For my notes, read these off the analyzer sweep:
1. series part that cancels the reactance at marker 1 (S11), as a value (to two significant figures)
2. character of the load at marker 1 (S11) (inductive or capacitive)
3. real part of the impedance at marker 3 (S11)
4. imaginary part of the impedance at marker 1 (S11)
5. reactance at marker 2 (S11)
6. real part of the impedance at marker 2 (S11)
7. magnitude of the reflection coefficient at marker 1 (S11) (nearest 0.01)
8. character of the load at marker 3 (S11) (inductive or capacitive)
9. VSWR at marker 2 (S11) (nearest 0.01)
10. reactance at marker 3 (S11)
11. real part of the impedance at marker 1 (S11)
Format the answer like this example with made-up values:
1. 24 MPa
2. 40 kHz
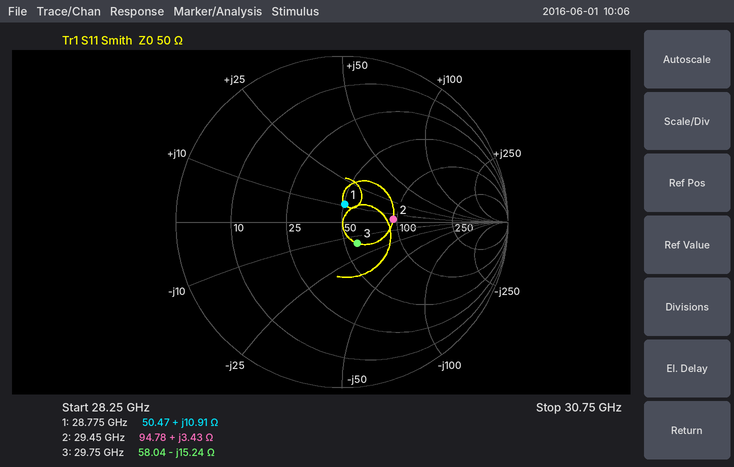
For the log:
1. 510 fF
2. inductive
3. 58.04 Ω
4. +10.91 Ω
5. +3.43 Ω
6. 94.78 Ω
7. 0.11
8. capacitive
9. 1.90
10. -15.24 Ω
11. 50.47 Ω
